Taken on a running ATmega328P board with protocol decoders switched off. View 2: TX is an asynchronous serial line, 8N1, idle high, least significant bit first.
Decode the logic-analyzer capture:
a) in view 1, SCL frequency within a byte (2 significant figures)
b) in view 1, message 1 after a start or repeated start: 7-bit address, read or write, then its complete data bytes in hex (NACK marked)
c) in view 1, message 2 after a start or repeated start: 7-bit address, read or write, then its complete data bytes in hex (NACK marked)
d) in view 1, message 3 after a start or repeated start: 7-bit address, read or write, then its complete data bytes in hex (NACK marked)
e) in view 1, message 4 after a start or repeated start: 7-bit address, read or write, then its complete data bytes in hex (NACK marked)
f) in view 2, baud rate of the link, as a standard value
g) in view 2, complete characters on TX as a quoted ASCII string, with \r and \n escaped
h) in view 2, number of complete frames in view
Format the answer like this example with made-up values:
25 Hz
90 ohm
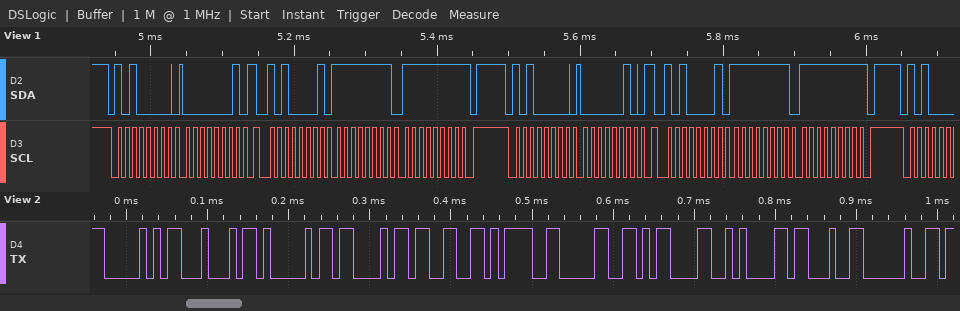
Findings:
100 kHz
0x50 write: 01
0x50 read: FF FF NACK
0x50 write: 02
0x50 read: FF FF NACK
115200 baud
"PDAC3=0\r\n# "
11
